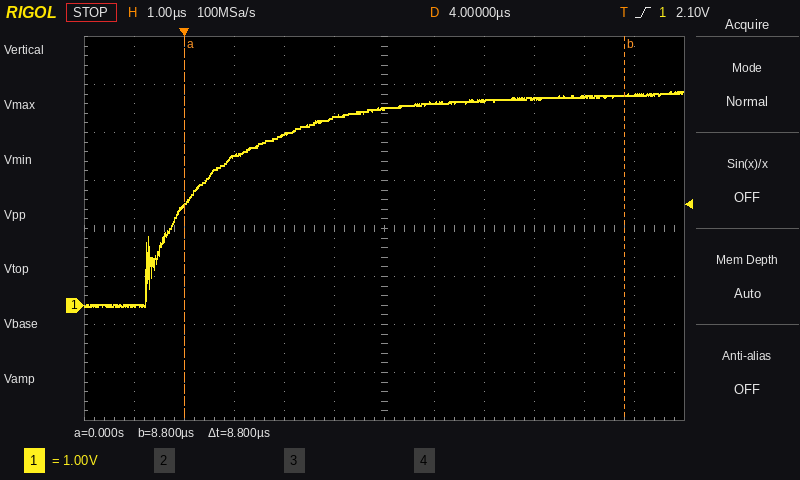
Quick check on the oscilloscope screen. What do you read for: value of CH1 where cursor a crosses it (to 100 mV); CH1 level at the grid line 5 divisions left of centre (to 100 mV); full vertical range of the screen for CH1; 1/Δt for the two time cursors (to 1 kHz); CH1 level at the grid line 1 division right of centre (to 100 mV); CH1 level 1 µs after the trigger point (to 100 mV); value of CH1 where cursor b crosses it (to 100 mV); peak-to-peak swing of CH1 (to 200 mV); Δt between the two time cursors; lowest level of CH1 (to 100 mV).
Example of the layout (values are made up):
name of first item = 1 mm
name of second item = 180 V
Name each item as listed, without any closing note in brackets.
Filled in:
value of CH1 where cursor a crosses it = 2.1 V
CH1 level at the grid line 5 divisions left of centre = 0.0 V
full vertical range of the screen for CH1 = 8 V
1/Δt for the two time cursors = 114 kHz
CH1 level at the grid line 1 division right of centre = 4.2 V
CH1 level 1 µs after the trigger point = 3.1 V
value of CH1 where cursor b crosses it = 4.4 V
peak-to-peak swing of CH1 = 4.4 V
Δt between the two time cursors = 8.8 µs
lowest level of CH1 = 0.0 V
